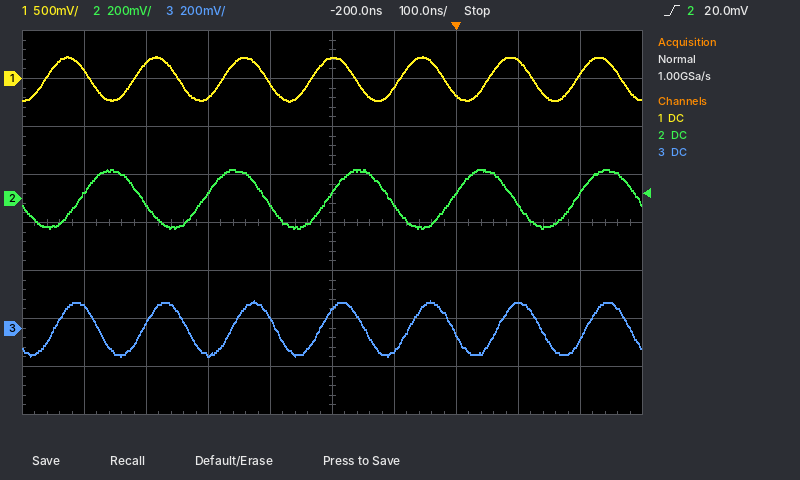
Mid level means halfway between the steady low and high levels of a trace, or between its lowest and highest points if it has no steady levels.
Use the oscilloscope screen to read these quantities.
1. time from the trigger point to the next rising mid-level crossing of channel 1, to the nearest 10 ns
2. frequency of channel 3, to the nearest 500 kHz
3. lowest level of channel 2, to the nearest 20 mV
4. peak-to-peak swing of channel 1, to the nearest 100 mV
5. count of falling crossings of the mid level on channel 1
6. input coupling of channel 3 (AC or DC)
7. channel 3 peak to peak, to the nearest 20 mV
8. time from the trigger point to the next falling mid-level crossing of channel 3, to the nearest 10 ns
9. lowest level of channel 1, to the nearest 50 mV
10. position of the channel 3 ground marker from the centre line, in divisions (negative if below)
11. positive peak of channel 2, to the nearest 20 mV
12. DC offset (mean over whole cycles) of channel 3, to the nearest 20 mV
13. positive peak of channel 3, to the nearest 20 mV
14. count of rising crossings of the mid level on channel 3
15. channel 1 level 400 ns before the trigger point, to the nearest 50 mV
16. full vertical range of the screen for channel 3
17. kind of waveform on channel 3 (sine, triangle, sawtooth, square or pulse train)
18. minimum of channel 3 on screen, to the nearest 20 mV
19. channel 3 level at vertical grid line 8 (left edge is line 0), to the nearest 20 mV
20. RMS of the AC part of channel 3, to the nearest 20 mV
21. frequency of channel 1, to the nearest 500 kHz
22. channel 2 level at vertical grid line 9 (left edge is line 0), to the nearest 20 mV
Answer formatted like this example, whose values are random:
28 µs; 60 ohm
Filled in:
50 ns; 7.0 MHz; -120 mV; 500 mV; 7; DC; 240 mV; 140 ns; -250 mV; -2.2 div; 120 mV; 0 mV; 120 mV; 7; -200 mV; 1.6 V; sine; -120 mV; 100 mV; 80 mV; 7.0 MHz; 20 mV
